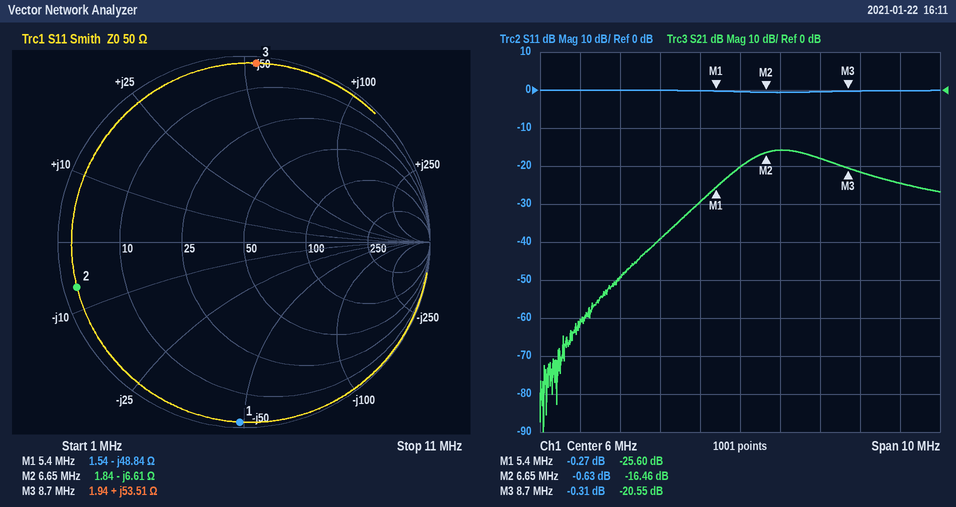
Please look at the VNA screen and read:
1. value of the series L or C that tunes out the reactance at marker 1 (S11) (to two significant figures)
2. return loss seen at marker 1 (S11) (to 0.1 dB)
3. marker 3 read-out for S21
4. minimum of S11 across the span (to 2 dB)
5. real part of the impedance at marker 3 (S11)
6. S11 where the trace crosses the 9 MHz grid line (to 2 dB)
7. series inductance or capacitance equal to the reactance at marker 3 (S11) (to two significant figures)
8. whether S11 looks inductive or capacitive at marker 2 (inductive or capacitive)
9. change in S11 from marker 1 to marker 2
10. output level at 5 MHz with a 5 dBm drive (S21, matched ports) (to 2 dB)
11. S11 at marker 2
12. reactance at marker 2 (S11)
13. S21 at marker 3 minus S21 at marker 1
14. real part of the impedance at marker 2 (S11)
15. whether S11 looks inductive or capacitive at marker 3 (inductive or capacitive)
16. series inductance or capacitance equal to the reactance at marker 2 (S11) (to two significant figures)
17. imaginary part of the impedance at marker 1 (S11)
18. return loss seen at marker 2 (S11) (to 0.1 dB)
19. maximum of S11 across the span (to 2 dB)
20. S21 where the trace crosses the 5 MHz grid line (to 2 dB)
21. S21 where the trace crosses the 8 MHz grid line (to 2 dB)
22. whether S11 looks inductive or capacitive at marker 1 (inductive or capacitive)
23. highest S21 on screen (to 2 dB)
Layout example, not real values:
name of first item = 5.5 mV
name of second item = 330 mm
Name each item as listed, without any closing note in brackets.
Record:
value of the series L or C that tunes out the reactance at marker 1 (S11) = 1.4 µH
return loss seen at marker 1 (S11) = 0.3 dB
marker 3 read-out for S21 = -20.55 dB
minimum of S11 across the span = 0 dB
real part of the impedance at marker 3 = 1.94 Ω
S11 where the trace crosses the 9 MHz grid line = 0 dB
series inductance or capacitance equal to the reactance at marker 3 (S11) = 980 nH
whether S11 looks inductive or capacitive at marker 2 = capacitive
change in S11 from marker 1 to marker 2 = -0.36 dB
output level at 5 MHz with a 5 dBm drive (S21, matched ports) = -24 dBm
S11 at marker 2 = -0.63 dB
reactance at marker 2 = -6.61 Ω
S21 at marker 3 minus S21 at marker 1 = 5.05 dB
real part of the impedance at marker 2 = 1.84 Ω
whether S11 looks inductive or capacitive at marker 3 = inductive
series inductance or capacitance equal to the reactance at marker 2 (S11) = 3.6 nF
imaginary part of the impedance at marker 1 = -48.84 Ω
return loss seen at marker 2 (S11) = 0.6 dB
maximum of S11 across the span = 0 dB
S21 where the trace crosses the 5 MHz grid line = -30 dB
S21 where the trace crosses the 8 MHz grid line = -18 dB
whether S11 looks inductive or capacitive at marker 1 = capacitive
highest S21 on screen = -16 dB
